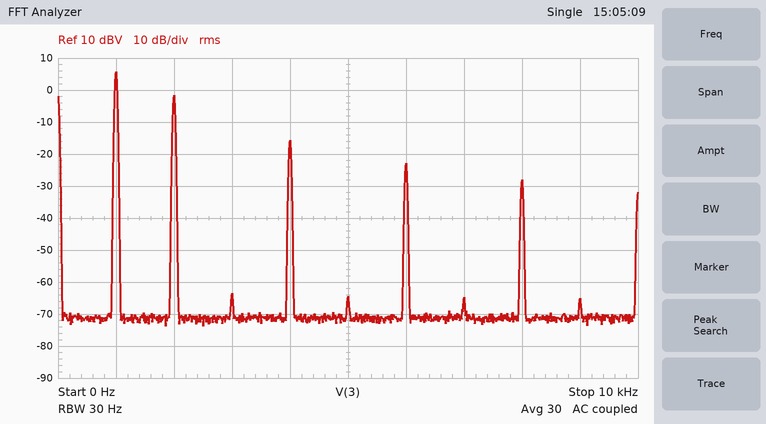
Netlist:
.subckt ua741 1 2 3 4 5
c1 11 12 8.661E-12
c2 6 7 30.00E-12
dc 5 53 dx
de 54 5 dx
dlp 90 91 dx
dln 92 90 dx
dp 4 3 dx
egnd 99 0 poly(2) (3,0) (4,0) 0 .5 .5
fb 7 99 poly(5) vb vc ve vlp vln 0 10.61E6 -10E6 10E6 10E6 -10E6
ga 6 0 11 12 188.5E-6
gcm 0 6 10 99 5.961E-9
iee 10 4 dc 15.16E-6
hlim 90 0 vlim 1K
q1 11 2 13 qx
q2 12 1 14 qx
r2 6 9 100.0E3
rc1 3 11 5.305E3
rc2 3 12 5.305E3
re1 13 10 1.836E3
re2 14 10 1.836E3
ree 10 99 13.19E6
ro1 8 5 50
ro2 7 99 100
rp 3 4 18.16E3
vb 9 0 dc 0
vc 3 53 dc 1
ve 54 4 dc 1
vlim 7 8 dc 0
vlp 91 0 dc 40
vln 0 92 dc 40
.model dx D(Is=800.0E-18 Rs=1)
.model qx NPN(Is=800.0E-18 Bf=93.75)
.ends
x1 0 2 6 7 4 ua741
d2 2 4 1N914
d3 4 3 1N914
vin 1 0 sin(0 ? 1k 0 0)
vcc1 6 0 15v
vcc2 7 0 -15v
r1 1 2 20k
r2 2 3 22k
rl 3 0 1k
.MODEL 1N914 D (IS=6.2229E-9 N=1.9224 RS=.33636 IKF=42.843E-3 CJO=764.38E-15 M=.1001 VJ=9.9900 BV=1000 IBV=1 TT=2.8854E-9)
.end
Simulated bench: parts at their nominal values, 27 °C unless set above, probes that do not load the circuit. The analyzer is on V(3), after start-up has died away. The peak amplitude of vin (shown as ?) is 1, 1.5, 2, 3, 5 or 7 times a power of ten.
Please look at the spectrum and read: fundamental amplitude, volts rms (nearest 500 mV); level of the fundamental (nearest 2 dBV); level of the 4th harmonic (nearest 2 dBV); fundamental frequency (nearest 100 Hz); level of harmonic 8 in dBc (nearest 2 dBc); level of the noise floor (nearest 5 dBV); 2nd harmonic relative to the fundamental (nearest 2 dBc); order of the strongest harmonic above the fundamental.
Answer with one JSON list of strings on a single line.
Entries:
["2.0 V", "6 dBV", "-16 dBV", "1.0 kHz", "-34 dBc", "-70 dBV", "-8 dBc", "2"]
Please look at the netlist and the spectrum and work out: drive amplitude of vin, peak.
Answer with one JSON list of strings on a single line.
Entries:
["5 V"]
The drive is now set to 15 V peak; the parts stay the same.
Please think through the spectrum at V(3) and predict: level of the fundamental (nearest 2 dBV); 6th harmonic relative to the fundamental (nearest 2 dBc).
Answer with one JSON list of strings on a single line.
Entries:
["14 dBV", "-34 dBc"]
